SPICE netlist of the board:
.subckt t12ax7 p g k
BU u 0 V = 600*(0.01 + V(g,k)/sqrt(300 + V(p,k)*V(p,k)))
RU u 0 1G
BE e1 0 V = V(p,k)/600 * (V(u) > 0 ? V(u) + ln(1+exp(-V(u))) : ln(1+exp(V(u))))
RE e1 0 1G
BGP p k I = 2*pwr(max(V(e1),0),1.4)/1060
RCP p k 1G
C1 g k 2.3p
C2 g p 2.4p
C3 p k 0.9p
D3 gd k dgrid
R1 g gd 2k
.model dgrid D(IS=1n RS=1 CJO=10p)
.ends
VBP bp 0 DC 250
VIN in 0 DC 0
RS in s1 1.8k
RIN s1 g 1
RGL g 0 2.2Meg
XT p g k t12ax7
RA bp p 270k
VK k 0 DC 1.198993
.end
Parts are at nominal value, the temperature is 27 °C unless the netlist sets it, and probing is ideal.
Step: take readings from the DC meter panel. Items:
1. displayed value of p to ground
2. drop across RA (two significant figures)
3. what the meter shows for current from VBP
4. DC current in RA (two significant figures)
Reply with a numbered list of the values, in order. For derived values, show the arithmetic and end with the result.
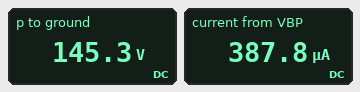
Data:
1. 145.3 V
2. 250 V - 145.3 V = 100 V
3. 387.8 µA
4. (250 V - 145.3 V) / 270 kΩ = 390 µA
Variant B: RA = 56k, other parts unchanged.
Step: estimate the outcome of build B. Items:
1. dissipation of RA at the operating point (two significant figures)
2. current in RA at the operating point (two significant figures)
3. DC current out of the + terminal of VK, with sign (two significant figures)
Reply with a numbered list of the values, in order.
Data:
1. 72 mW
2. 1.1 mA
3. -1.1 mA
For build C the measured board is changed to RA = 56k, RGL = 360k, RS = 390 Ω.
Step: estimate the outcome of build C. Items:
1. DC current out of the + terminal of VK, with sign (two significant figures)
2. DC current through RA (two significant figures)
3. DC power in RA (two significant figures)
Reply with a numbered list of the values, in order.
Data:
1. -1.1 mA
2. 1.1 mA
3. 72 mW
